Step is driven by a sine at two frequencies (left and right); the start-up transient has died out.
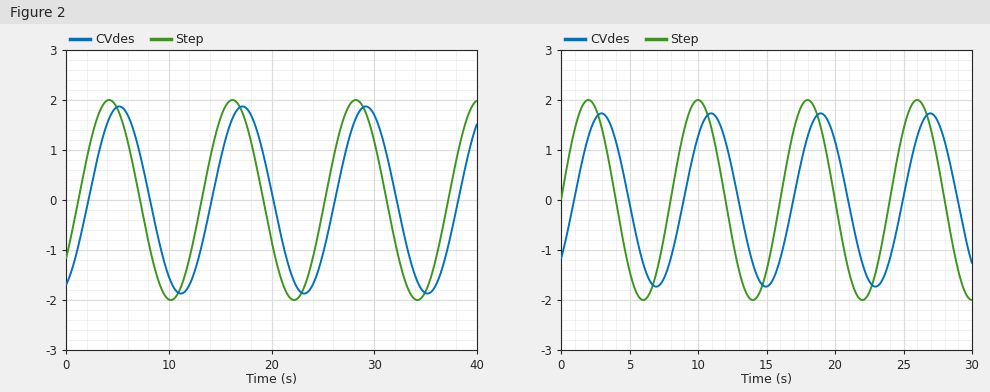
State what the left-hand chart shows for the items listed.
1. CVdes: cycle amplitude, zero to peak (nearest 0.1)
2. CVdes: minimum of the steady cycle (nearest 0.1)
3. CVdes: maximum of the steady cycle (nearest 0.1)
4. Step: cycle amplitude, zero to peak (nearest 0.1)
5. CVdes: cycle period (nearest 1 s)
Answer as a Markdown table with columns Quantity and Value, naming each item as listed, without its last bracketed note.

| Quantity | Value |
|---|---|
| CVdes: cycle amplitude, zero to peak | 1.9 |
| CVdes: minimum of the steady cycle | -1.9 |
| CVdes: maximum of the steady cycle | 1.9 |
| Step: cycle amplitude, zero to peak | 2.0 |
| CVdes: cycle period | 12 s |
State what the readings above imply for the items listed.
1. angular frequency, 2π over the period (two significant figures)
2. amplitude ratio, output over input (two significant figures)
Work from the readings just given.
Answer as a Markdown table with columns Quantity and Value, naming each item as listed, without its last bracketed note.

| Quantity | Value |
|---|---|
| angular frequency, 2π over the period | 0.52 rad/s |
| amplitude ratio, output over input | 0.95 |
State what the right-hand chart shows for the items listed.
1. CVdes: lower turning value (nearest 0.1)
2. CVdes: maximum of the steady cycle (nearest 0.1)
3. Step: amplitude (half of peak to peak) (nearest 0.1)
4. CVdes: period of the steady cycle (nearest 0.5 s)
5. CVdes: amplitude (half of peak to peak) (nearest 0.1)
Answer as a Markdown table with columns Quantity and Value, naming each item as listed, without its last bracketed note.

| Quantity | Value |
|---|---|
| CVdes: lower turning value | -1.7 |
| CVdes: maximum of the steady cycle | 1.7 |
| Step: amplitude (half of peak to peak) | 2.0 |
| CVdes: period of the steady cycle | 8.0 s |
| CVdes: amplitude (half of peak to peak) | 1.7 |
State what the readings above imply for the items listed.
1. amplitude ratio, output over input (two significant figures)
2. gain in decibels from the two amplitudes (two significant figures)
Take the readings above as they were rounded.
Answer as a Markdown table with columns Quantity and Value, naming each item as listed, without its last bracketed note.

| Quantity | Value |
|---|---|
| amplitude ratio, output over input | 0.85 |
| gain in decibels from the two amplitudes | -1.4 dB |
